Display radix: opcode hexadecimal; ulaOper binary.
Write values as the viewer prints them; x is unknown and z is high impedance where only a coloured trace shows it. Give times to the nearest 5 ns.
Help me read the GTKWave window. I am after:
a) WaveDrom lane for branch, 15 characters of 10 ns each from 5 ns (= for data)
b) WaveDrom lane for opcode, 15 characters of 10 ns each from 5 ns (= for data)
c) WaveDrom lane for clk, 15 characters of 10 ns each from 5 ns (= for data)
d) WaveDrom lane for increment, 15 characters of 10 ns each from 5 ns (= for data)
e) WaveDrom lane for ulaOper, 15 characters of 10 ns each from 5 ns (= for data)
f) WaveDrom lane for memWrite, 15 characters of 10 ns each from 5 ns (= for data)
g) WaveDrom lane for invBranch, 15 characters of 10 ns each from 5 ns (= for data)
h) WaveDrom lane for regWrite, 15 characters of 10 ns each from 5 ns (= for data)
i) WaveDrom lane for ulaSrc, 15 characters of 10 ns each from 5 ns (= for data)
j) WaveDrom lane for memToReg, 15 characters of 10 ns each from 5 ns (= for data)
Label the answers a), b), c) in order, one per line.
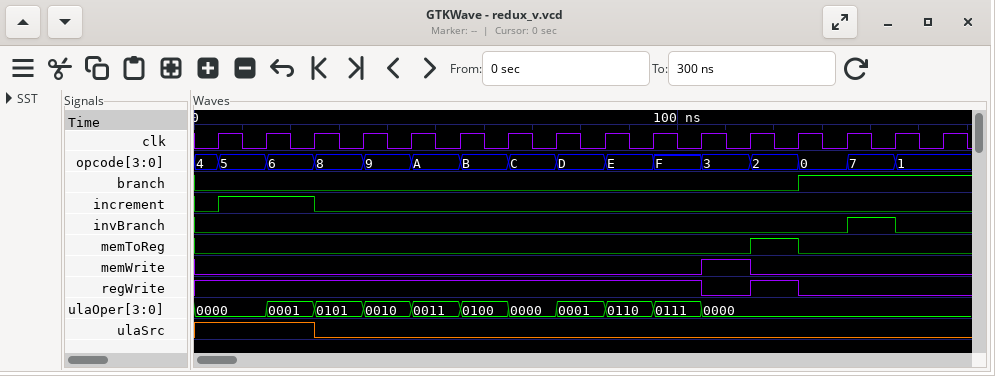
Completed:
a) {name: 'branch', wave: '0...........1..'}
b) {name: 'opcode', wave: '===============', data: '5 6 8 9 A B C D E F 3 2 0 7 1'}
c) {name: 'clk', wave: 'p..............'}
d) {name: 'increment', wave: '1.0............'}
e) {name: 'ulaOper', wave: '===========....', data: '0000 0001 0101 0010 0011 0100 0000 0001 0110 0111 0000'}
f) {name: 'memWrite', wave: '0.........10...'}
g) {name: 'invBranch', wave: '0............10'}
h) {name: 'regWrite', wave: '1.........010..'}
i) {name: 'ulaSrc', wave: '1.0............'}
j) {name: 'memToReg', wave: '0..........10..'}
